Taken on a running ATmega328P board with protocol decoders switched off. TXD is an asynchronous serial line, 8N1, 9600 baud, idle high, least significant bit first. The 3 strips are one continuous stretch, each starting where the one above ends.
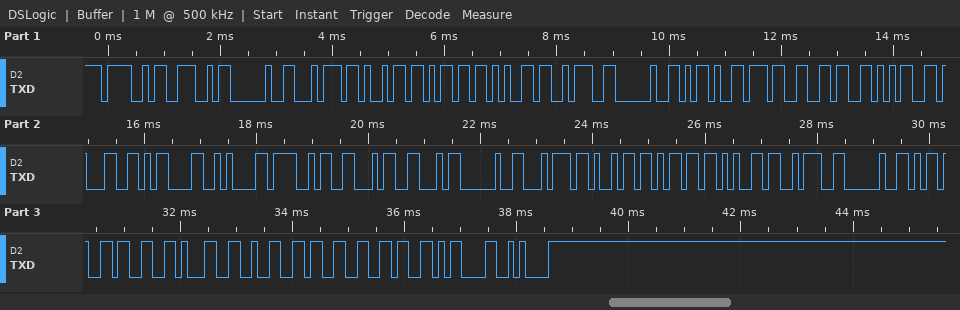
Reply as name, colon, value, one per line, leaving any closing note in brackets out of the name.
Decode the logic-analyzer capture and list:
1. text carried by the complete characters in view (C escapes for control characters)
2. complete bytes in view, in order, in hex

text carried by the complete characters in view: "ON time: -7651\r\nOFF time: -31236\r\n"
complete bytes in view, in order, in hex: 4F 4E 20 74 69 6D 65 3A 20 2D 37 36 35 31 0D 0A 4F 46 46 20 74 69 6D 65 3A 20 2D 33 31 32 33 36 0D 0A
